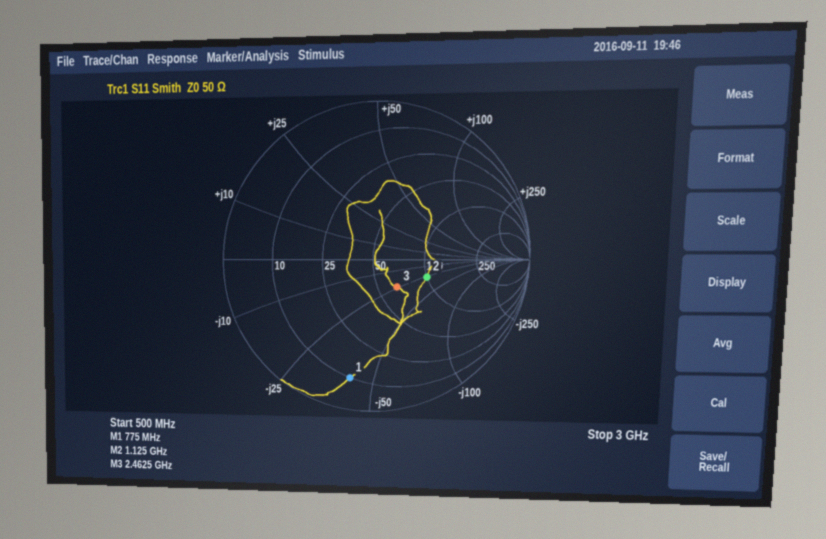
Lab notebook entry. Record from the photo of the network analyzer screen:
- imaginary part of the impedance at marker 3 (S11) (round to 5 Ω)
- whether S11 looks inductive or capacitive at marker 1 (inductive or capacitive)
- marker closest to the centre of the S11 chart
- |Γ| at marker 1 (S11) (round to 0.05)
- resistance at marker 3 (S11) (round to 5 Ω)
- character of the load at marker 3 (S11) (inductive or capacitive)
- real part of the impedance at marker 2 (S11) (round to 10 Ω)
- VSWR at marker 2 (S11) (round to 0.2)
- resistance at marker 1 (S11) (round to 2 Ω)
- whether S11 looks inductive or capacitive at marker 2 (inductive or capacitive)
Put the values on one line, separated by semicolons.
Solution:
-25 Ω; capacitive; marker 3; 0.80; 65 Ω; capacitive; 100 Ω; 2.2; 10 Ω; capacitive
